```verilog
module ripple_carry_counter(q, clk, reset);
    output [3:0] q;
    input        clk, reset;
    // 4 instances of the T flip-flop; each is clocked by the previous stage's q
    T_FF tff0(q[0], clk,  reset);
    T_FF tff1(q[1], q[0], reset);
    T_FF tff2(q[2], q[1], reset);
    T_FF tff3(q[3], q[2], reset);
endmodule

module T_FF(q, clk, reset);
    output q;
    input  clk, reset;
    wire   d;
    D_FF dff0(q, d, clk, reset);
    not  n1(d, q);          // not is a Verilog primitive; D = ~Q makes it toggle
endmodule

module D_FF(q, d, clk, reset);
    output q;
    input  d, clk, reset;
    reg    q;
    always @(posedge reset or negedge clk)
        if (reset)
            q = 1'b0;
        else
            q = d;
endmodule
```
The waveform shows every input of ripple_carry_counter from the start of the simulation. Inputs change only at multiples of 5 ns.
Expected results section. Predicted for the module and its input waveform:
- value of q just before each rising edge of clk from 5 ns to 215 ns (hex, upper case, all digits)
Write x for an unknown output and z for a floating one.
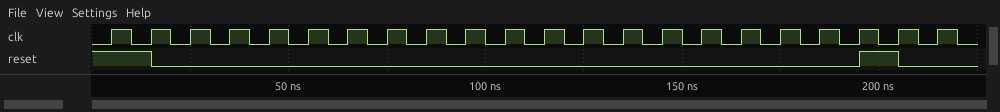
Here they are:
0, 0, 1, 2, 3, 4, 5, 6, 7, 8, 9, A, B, C, D, E, F, 0, 1, 2, 0, 1
